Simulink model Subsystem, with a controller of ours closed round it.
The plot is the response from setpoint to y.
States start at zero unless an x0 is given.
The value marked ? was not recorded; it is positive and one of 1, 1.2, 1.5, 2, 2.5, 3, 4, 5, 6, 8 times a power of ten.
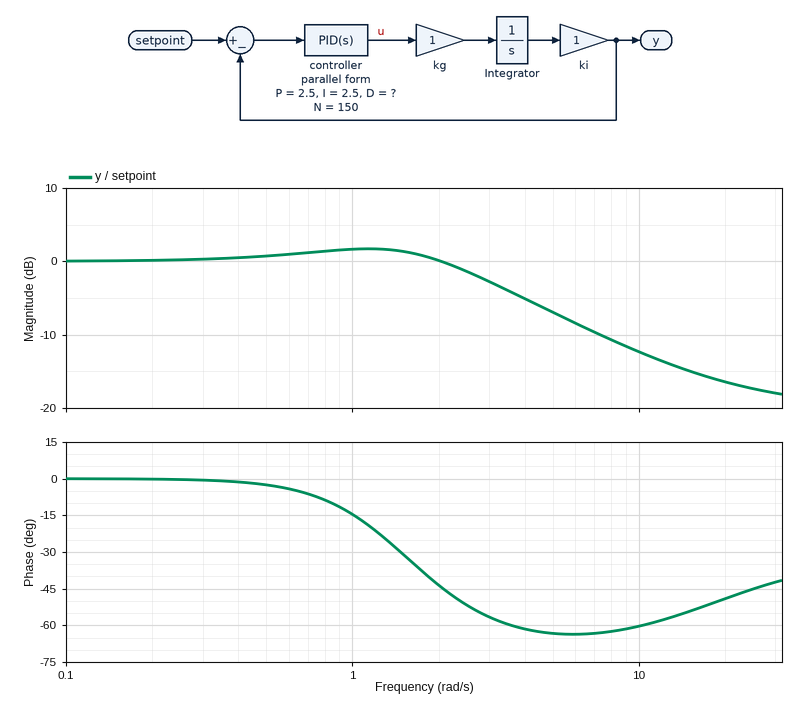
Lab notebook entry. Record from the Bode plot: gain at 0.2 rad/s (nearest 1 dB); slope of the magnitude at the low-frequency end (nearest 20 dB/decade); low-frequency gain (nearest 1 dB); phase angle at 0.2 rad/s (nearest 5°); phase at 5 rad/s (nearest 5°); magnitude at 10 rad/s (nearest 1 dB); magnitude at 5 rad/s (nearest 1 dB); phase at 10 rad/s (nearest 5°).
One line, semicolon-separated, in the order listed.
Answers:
0 dB; 0 dB/decade; 0 dB; 0°; -65°; -12 dB; -7 dB; -60°
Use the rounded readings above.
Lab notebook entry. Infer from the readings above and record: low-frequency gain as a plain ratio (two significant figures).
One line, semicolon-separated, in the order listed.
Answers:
1.0
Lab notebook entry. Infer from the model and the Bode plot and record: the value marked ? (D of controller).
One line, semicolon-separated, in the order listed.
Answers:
0.1
